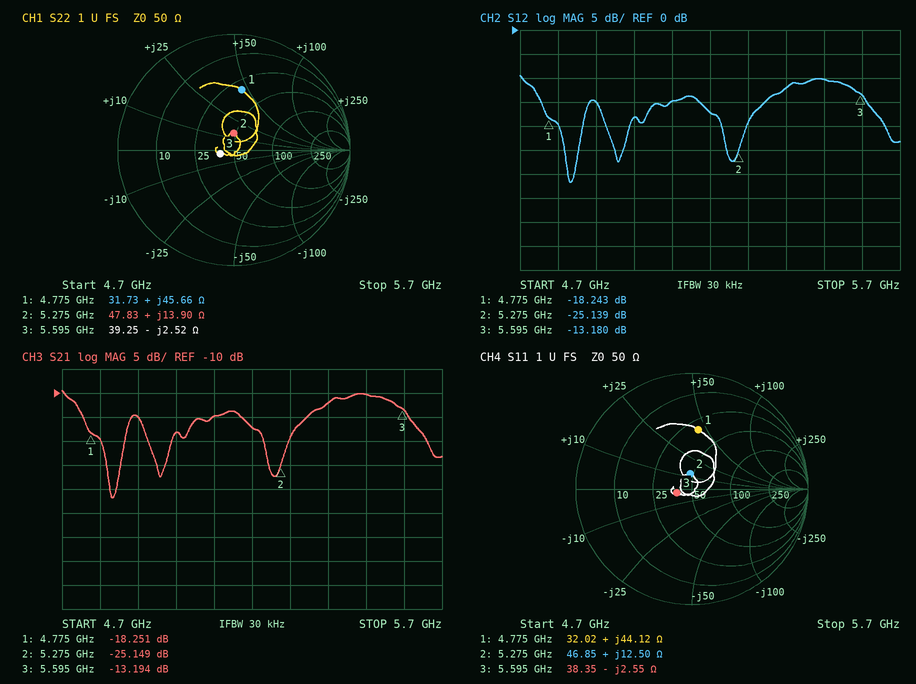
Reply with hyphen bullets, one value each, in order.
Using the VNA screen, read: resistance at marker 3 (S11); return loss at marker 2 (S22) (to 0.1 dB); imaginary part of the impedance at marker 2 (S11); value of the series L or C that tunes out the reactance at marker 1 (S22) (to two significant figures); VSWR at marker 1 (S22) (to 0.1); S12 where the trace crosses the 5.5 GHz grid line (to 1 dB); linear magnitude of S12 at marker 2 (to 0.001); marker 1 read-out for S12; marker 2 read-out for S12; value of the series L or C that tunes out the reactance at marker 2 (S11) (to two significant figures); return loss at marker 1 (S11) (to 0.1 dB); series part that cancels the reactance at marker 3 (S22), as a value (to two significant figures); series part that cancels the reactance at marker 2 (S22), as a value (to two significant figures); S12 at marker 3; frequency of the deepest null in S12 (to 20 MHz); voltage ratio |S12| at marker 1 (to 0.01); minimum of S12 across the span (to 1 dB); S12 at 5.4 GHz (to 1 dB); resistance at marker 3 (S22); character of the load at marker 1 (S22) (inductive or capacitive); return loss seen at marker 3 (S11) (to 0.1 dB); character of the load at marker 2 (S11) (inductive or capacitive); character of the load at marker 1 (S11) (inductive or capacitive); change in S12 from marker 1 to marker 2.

- 38.35 Ω
- 16.9 dB
- +12.50 Ω
- 730 fF
- 3.2
- -10 dB
- 0.055
- -18.243 dB
- -25.139 dB
- 2.4 pF
- 5.8 dB
- 72 pH
- 2.2 pF
- -13.180 dB
- 4.84 GHz
- 0.12
- -32 dB
- -12 dB
- 39.25 Ω
- inductive
- 17.4 dB
- inductive
- inductive
- -6.896 dB
